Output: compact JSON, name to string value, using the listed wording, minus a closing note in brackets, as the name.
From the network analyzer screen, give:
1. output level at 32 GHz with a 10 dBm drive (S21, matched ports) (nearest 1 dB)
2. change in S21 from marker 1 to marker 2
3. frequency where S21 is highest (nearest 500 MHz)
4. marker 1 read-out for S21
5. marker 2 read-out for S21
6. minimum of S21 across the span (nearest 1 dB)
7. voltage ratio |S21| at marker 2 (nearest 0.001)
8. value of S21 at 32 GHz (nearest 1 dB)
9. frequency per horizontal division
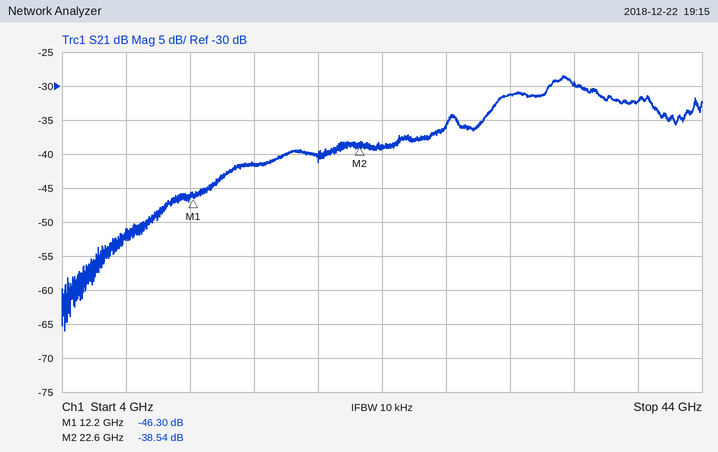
{"output level at 32 GHz with a 10 dBm drive (S21, matched ports)": "-21 dBm", "change in S21 from marker 1 to marker 2": "7.76 dB", "frequency where S21 is highest": "35.5 GHz", "marker 1 read-out for S21": "-46.30 dB", "marker 2 read-out for S21": "-38.54 dB", "minimum of S21 across the span": "-66 dB", "voltage ratio |S21| at marker 2": "0.012", "value of S21 at 32 GHz": "-31 dB", "frequency per horizontal division": "4 GHz"}
